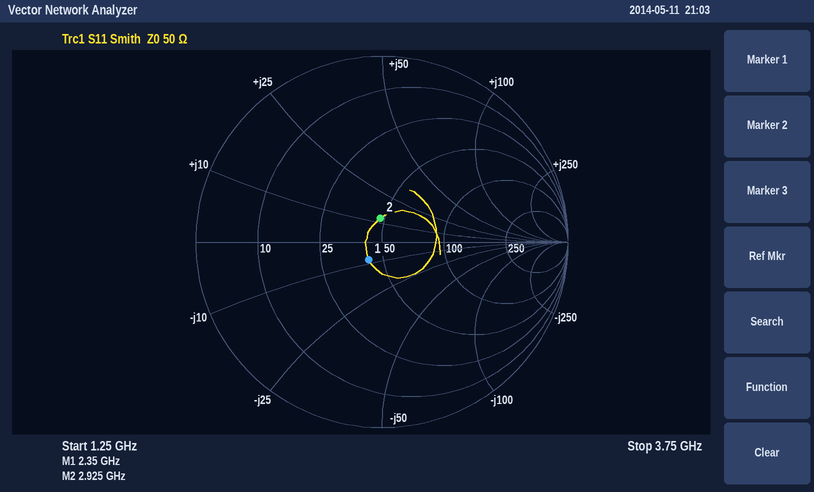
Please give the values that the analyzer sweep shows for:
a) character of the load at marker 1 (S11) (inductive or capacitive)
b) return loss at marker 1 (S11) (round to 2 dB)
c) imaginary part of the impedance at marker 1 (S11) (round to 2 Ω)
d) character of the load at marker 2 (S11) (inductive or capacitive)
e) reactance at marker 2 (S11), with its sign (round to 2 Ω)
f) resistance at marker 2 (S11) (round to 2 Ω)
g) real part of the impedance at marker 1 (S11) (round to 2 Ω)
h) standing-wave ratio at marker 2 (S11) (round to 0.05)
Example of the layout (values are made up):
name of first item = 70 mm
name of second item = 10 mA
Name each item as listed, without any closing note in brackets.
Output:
character of the load at marker 1 (S11) = capacitive
return loss at marker 1 (S11) = 18 dB
imaginary part of the impedance at marker 1 (S11) = -8 Ω
character of the load at marker 2 (S11) = inductive
reactance at marker 2 (S11), with its sign = +12 Ω
resistance at marker 2 (S11) = 48 Ω
real part of the impedance at marker 1 (S11) = 42 Ω
standing-wave ratio at marker 2 (S11) = 1.30
